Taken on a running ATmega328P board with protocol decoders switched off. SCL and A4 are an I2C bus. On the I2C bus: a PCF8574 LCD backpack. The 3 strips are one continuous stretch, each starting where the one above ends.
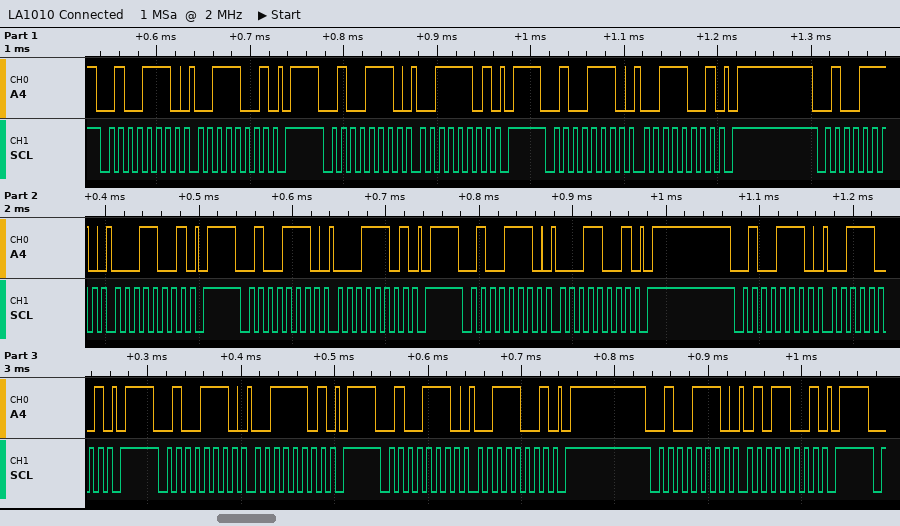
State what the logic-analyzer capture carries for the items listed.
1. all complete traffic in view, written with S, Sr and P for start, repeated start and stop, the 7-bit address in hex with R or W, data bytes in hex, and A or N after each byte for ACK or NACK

S 27W A 39 A P S 27W A 3D A P S 27W A 39 A P S 27W A 19 A P S 27W A 1D A P S 27W A 19 A P S 27W A 39 A P S 27W A 3D A P S 27W A 39 A P S 27W A 59 A P
